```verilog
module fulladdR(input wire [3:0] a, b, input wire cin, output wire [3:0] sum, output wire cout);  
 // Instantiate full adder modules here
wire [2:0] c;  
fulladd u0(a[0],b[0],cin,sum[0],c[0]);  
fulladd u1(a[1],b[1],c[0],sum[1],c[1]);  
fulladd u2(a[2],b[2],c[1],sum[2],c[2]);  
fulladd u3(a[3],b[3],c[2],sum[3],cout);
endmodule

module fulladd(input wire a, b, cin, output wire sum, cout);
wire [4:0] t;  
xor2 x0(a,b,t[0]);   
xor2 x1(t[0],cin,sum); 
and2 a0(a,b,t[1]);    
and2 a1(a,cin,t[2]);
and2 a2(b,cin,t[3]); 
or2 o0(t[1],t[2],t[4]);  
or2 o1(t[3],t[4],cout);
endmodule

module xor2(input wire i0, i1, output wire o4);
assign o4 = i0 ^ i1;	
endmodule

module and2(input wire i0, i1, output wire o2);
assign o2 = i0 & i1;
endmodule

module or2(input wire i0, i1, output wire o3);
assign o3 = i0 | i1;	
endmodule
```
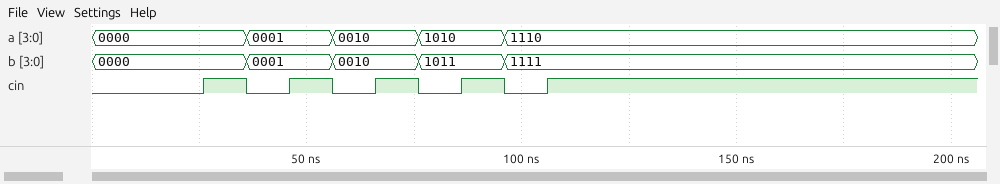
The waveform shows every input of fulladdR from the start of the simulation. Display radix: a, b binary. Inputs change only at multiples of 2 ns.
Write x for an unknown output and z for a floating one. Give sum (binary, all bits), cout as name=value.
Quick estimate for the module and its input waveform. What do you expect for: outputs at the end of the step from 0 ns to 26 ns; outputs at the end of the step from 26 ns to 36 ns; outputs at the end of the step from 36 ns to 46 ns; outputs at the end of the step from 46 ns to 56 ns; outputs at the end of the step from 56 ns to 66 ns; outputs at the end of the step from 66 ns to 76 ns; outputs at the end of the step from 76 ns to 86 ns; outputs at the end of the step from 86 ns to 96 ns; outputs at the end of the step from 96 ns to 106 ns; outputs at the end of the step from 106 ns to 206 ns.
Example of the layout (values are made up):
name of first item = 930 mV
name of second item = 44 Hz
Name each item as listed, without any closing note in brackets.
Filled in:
outputs at the end of the step from 0 ns to 26 ns = sum=0000, cout=0
outputs at the end of the step from 26 ns to 36 ns = sum=0001, cout=0
outputs at the end of the step from 36 ns to 46 ns = sum=0010, cout=0
outputs at the end of the step from 46 ns to 56 ns = sum=0011, cout=0
outputs at the end of the step from 56 ns to 66 ns = sum=0100, cout=0
outputs at the end of the step from 66 ns to 76 ns = sum=0101, cout=0
outputs at the end of the step from 76 ns to 86 ns = sum=0101, cout=1
outputs at the end of the step from 86 ns to 96 ns = sum=0110, cout=1
outputs at the end of the step from 96 ns to 106 ns = sum=1101, cout=1
outputs at the end of the step from 106 ns to 206 ns = sum=1110, cout=1
